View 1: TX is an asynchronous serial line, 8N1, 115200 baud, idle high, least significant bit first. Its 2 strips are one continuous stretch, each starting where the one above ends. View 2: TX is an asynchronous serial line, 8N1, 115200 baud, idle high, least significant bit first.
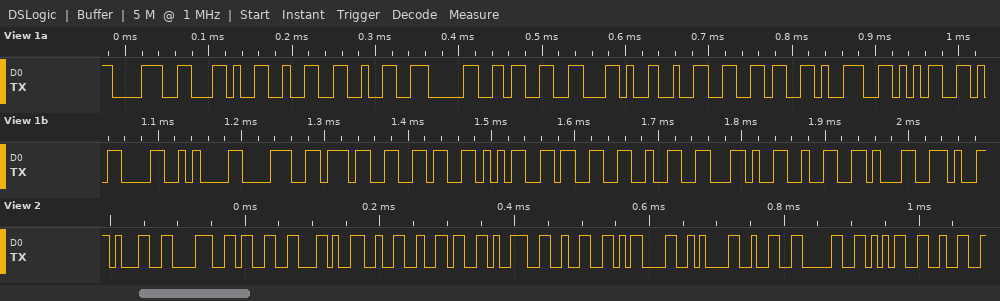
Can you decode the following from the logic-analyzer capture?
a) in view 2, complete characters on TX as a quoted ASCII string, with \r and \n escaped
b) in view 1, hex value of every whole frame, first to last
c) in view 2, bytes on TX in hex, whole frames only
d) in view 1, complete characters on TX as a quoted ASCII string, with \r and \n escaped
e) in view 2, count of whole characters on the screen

"183,2692\r\n2052"
0x38 0x2C 0x32 0x32 0x30 0x33 0x2C 0x32 0x36 0x39 0x35 0x0D 0x0A 0x38 0x37 0x36 0x35 0x33 0x32 0x2C 0x32 0x31
31 38 33 2C 32 36 39 32 0D 0A 32 30 35 32
"8,2203,2695\r\n876532,21"
14
